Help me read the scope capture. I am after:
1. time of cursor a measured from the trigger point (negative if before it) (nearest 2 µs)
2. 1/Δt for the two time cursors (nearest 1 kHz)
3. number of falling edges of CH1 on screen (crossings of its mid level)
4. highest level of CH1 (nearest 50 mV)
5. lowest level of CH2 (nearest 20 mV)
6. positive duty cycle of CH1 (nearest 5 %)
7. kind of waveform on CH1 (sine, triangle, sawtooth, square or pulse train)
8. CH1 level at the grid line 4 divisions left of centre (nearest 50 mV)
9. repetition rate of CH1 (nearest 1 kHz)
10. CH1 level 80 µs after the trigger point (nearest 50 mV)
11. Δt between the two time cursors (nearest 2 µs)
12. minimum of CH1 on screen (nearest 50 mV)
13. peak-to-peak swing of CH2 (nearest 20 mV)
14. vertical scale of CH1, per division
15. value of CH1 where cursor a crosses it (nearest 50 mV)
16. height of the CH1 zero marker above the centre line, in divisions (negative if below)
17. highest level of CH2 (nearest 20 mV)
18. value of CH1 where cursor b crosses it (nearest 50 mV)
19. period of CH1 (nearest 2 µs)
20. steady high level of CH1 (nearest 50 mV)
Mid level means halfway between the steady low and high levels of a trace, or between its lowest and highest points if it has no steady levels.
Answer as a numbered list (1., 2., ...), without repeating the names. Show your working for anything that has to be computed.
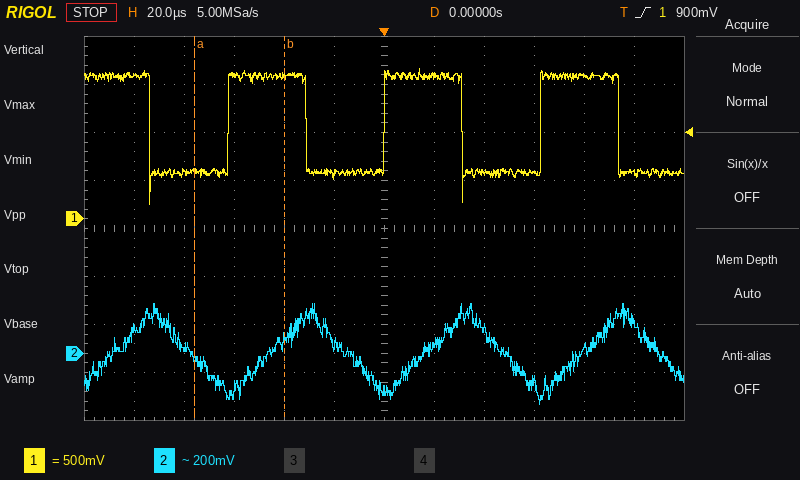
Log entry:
1. -76 µs
2. 1 / 36 µs ≈ 28 kHz
3. 4
4. 1.55 V
5. -220 mV
6. 50 %
7. square
8. 500 mV
9. 1 / 62 µs ≈ 16 kHz
10. 1.50 V
11. 36 µs
12. 150 mV
13. 200 mV − (-220 mV) = 420 mV
14. 500 mV
15. 500 mV
16. +0.2 div
17. 200 mV
18. 1.50 V
19. 62 µs
20. 1.50 V
